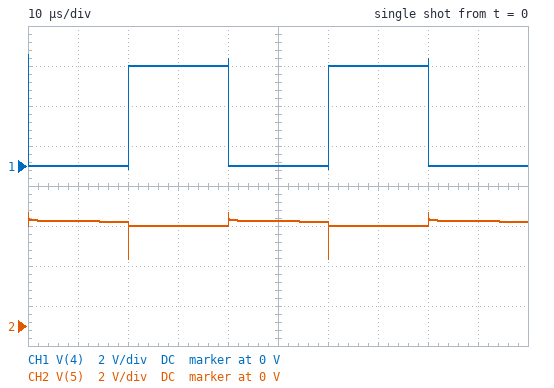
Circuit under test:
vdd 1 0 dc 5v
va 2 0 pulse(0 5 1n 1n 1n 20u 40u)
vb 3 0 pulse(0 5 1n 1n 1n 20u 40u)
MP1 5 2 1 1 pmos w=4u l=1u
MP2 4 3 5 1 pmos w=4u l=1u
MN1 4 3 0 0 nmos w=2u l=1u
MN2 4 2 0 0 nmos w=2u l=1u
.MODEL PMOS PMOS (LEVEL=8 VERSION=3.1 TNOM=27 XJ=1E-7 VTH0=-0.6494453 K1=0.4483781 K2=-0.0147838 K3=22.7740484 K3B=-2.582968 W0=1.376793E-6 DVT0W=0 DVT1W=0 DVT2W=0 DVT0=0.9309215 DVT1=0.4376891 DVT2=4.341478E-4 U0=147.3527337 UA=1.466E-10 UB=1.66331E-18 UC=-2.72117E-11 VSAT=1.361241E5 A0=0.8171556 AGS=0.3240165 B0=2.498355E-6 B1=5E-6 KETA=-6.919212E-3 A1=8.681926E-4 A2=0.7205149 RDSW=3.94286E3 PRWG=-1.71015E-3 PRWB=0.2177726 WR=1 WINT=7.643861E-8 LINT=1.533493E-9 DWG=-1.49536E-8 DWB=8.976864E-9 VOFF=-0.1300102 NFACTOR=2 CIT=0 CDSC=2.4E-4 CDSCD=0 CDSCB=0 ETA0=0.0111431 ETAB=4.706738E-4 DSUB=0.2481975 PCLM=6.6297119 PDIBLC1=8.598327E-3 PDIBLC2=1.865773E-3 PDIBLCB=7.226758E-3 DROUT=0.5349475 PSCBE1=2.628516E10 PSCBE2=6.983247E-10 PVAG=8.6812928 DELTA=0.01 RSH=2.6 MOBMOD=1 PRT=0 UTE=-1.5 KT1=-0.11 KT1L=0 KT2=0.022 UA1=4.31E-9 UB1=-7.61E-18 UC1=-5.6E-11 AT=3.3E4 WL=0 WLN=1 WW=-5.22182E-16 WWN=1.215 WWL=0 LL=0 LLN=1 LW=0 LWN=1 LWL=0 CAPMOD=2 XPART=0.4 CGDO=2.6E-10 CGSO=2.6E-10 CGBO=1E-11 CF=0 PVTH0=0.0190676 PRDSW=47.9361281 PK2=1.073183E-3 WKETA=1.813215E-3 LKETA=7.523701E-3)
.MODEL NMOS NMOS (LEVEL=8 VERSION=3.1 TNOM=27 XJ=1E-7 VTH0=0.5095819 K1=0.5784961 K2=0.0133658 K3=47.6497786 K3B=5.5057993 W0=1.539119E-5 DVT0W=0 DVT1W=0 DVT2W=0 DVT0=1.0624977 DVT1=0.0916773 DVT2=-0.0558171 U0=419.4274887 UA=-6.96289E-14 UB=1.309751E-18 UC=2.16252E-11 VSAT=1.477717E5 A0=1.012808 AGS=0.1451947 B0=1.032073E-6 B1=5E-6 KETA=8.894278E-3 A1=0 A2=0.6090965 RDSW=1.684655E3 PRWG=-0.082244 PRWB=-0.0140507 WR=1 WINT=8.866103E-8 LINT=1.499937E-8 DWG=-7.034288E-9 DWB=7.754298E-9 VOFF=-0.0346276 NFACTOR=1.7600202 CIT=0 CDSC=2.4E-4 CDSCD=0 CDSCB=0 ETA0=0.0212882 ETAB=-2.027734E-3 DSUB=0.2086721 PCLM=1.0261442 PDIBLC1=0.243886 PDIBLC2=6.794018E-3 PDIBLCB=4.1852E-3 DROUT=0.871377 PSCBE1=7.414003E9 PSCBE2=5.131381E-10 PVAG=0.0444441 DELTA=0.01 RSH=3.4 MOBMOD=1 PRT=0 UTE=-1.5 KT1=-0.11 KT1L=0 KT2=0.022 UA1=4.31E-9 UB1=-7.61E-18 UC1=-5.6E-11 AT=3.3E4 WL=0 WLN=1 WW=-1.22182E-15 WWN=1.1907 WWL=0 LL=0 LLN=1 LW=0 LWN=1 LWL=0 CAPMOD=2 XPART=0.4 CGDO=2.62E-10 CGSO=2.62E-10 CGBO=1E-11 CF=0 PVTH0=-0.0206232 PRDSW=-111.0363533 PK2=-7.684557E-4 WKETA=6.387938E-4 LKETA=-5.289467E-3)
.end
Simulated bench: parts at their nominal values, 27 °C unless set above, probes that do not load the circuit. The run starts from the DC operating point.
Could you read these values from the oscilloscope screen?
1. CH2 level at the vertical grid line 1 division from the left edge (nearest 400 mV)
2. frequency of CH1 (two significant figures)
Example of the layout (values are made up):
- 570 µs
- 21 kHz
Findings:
- 5.2 V
- 25 kHz
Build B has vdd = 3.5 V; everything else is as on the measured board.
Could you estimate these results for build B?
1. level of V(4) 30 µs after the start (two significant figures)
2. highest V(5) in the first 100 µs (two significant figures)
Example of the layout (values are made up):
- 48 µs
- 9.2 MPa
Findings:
- 3.5 V
- 4.9 V
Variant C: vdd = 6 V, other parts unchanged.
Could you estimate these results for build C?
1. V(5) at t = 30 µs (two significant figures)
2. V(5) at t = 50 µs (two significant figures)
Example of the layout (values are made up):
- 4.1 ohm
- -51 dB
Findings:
- 6.0 V
- 5.9 V
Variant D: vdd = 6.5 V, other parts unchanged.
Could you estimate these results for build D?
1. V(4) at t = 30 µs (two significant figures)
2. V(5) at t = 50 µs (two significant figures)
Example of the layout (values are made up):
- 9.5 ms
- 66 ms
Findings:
- 6.5 V
- 6.2 V
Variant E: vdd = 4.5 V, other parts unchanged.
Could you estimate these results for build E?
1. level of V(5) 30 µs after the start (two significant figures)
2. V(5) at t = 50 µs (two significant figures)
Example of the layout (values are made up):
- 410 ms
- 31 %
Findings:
- 4.5 V
- 5.1 V
